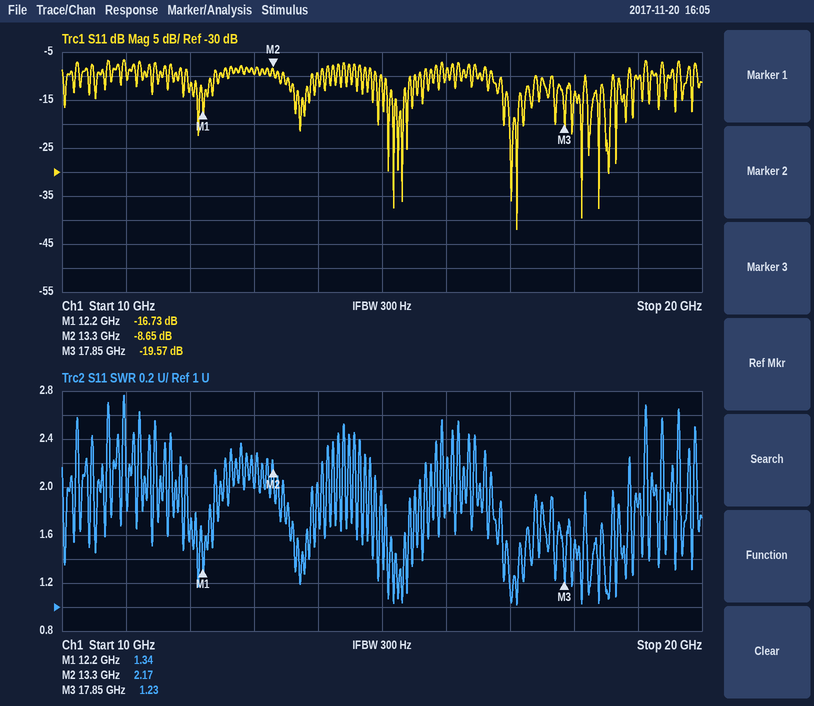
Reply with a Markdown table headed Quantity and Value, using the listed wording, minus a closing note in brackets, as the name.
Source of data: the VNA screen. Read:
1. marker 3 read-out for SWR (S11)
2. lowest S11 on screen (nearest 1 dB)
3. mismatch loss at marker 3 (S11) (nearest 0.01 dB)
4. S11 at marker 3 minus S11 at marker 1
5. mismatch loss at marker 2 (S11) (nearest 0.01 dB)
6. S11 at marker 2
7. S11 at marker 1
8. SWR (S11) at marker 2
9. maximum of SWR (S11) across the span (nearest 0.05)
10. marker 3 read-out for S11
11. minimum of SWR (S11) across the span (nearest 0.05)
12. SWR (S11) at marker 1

| Quantity | Value |
|---|---|
| marker 3 read-out for SWR | 1.23 |
| lowest S11 on screen | -42 dB |
| mismatch loss at marker 3 (S11) | 0.05 dB |
| S11 at marker 3 minus S11 at marker 1 | -2.84 dB |
| mismatch loss at marker 2 (S11) | 0.64 dB |
| S11 at marker 2 | -8.65 dB |
| S11 at marker 1 | -16.73 dB |
| SWR (S11) at marker 2 | 2.17 |
| maximum of SWR (S11) across the span | 2.75 |
| marker 3 read-out for S11 | -19.57 dB |
| minimum of SWR (S11) across the span | 1.00 |
| SWR (S11) at marker 1 | 1.34 |
